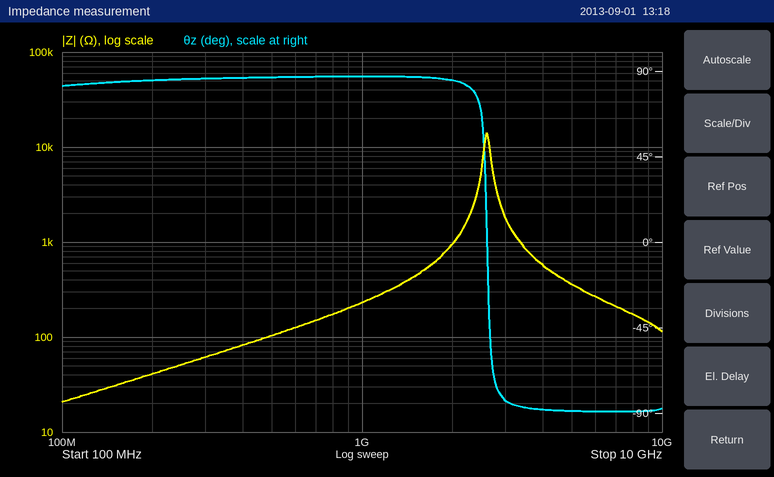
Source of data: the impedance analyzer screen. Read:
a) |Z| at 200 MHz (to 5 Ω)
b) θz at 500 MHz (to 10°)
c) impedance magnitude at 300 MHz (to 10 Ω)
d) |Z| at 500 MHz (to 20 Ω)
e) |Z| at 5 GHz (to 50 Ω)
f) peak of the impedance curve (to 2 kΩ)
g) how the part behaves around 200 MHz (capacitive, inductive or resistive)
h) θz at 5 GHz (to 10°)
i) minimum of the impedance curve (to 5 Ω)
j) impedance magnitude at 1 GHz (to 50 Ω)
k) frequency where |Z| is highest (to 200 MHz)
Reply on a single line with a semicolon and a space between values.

40 Ω; 90°; 60 Ω; 100 Ω; 350 Ω; 14 kΩ; inductive; -90°; 20 Ω; 250 Ω; 2.6 GHz
